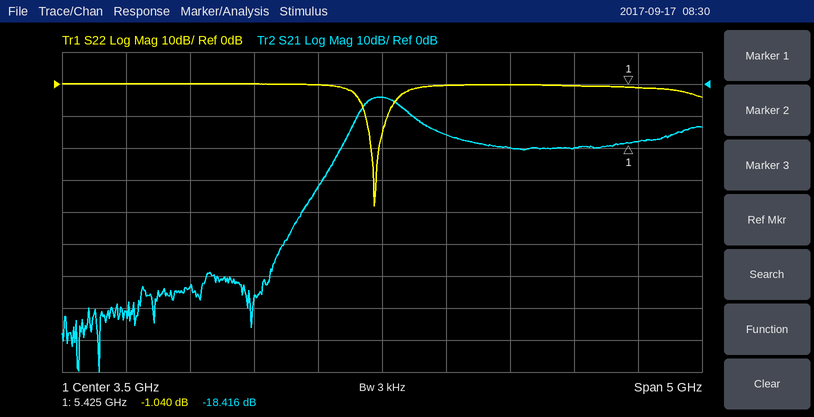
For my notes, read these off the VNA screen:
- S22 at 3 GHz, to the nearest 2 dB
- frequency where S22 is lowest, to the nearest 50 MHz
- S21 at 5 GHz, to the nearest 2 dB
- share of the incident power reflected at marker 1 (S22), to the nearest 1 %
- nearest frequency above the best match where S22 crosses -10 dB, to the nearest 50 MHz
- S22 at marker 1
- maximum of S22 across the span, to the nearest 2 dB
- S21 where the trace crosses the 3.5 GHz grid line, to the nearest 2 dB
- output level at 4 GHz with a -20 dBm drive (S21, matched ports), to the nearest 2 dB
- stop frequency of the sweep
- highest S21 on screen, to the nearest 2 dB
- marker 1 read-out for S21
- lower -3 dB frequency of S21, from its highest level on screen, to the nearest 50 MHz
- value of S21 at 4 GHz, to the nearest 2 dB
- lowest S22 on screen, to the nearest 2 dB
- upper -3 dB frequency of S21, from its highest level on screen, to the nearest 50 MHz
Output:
0 dB
3.45 GHz
-20 dB
79 %
3.55 GHz
-1.040 dB
0 dB
-4 dB
-36 dBm
6 GHz
-4 dB
-18.416 dB
3.35 GHz
-16 dB
-38 dB
3.65 GHz
